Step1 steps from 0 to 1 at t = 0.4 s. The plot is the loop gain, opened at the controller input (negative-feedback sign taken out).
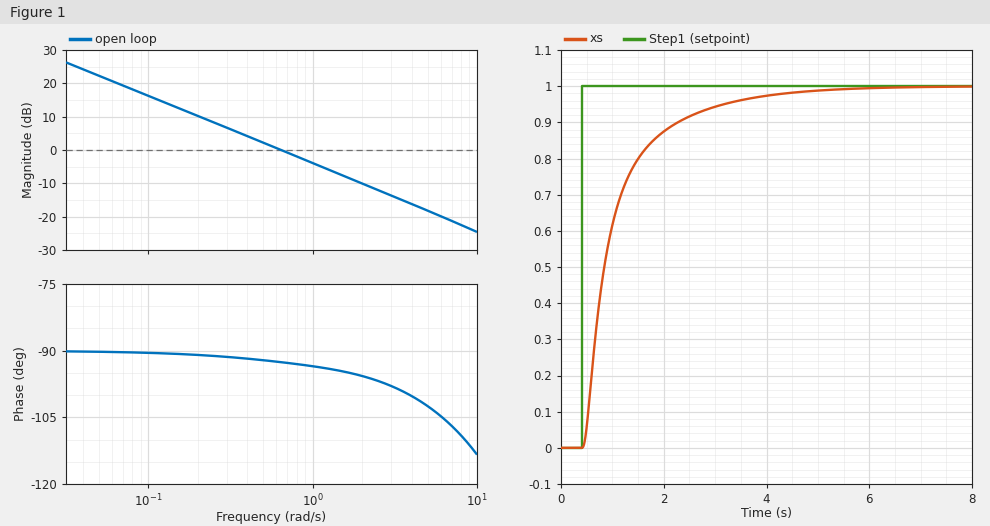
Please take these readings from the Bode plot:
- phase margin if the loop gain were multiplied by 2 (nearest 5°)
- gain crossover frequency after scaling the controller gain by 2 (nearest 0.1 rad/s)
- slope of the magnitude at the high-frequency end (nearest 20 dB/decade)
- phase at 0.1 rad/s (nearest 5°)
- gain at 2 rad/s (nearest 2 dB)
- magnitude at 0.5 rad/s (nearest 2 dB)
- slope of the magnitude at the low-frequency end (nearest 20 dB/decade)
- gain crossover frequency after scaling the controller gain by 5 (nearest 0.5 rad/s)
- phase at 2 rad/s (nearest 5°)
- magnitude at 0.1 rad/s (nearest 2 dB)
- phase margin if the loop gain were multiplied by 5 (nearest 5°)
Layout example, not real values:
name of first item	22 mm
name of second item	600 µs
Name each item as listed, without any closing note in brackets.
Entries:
phase margin if the loop gain were multiplied by 2	85°
gain crossover frequency after scaling the controller gain by 2	1.3 rad/s
slope of the magnitude at the high-frequency end	-20 dB/decade
phase at 0.1 rad/s	-90°
gain at 2 rad/s	-10 dB
magnitude at 0.5 rad/s	2 dB
slope of the magnitude at the low-frequency end	-20 dB/decade
gain crossover frequency after scaling the controller gain by 5	3.0 rad/s
phase at 2 rad/s	-95°
magnitude at 0.1 rad/s	16 dB
phase margin if the loop gain were multiplied by 5	80°
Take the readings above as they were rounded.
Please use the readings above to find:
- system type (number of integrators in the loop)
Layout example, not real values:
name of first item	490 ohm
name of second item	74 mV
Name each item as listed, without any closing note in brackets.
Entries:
system type	1
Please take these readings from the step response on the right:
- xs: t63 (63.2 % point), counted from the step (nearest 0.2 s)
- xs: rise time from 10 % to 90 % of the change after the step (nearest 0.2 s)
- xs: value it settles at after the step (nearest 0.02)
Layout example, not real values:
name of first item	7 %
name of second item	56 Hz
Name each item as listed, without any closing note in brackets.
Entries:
xs: t63 (63.2 % point), counted from the step	0.6 s
xs: rise time from 10 % to 90 % of the change after the step	1.8 s
xs: value it settles at after the step	1.00
